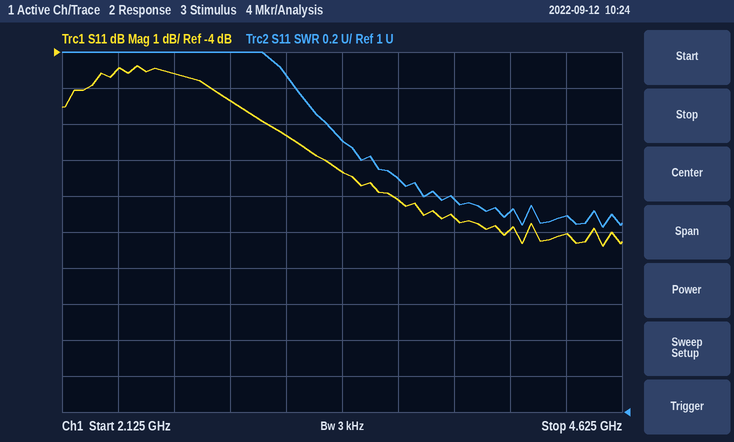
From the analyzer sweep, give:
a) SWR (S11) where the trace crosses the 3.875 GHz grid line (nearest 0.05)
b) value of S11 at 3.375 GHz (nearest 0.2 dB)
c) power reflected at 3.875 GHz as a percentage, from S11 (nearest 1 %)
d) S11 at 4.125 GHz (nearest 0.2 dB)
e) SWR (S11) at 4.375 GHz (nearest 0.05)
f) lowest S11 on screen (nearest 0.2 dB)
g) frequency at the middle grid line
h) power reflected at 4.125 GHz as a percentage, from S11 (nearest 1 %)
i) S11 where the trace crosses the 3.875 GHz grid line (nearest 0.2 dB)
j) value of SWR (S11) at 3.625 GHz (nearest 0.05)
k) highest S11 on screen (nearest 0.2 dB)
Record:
2.20
-7.4 dB
14 %
-9.0 dB
2.10
-9.4 dB
3.375 GHz
13 %
-8.6 dB
2.30
-4.4 dB
